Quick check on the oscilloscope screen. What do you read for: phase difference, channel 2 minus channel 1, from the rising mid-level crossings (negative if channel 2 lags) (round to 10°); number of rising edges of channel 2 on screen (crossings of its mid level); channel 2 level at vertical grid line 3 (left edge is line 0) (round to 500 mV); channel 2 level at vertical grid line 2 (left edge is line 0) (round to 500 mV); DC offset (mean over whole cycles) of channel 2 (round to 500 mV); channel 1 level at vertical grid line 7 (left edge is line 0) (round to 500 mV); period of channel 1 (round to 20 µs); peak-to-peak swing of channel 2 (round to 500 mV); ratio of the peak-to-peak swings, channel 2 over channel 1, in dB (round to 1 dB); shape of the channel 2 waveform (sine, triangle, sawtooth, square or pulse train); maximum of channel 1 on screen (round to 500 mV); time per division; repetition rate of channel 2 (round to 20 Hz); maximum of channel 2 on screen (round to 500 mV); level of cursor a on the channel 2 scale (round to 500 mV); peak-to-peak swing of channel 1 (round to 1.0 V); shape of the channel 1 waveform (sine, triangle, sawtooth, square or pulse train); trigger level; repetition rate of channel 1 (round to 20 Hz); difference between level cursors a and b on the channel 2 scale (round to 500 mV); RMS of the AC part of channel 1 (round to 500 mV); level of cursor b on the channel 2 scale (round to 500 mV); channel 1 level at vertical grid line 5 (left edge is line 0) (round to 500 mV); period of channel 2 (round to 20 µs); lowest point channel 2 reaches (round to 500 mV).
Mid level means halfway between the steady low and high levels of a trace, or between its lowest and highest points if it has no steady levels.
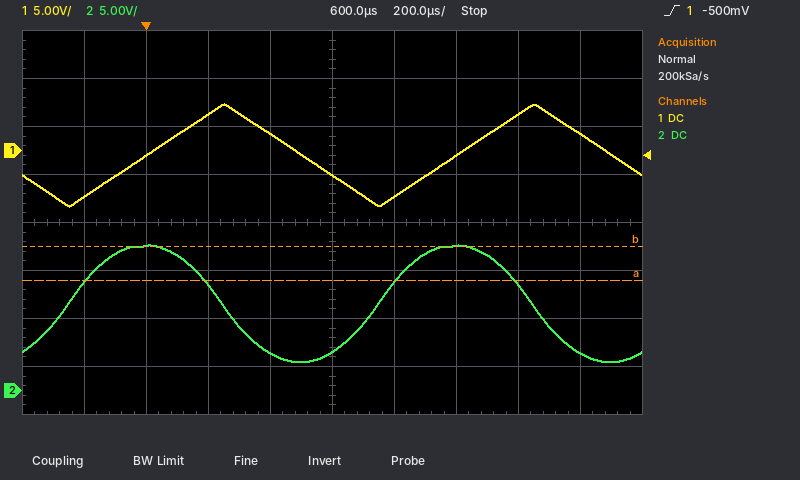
+90°
2
11.0 V
15.0 V
9.0 V
-500 mV
1.00 ms
12.0 V
1 dB
sine
5.0 V
200 µs
1.00 kHz
15.0 V
11.5 V
11.0 V
triangle
-500 mV
1.00 kHz
3.5 V
3.0 V
15.0 V
-2.5 V
1.00 ms
3.0 V
